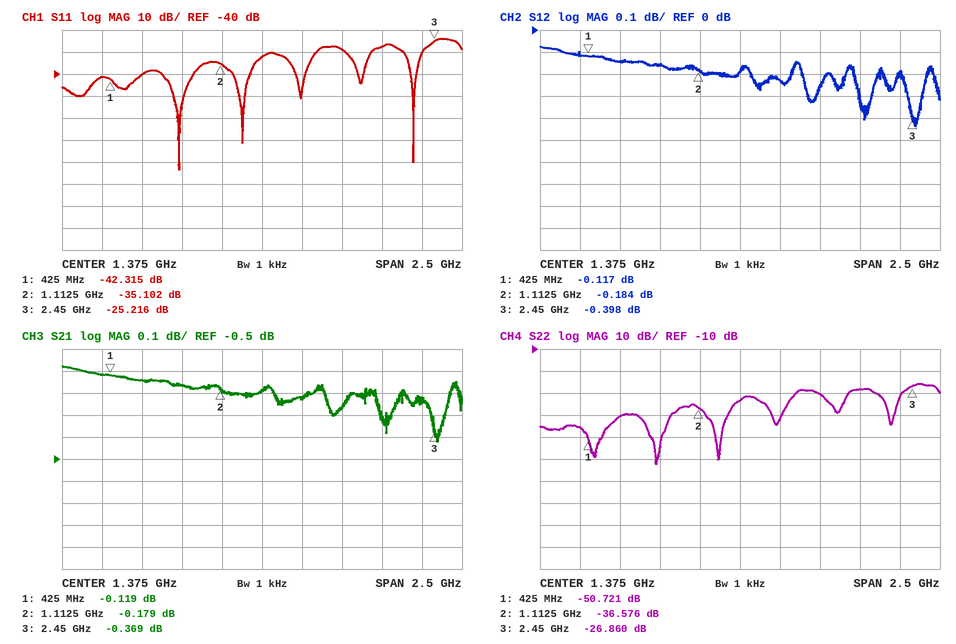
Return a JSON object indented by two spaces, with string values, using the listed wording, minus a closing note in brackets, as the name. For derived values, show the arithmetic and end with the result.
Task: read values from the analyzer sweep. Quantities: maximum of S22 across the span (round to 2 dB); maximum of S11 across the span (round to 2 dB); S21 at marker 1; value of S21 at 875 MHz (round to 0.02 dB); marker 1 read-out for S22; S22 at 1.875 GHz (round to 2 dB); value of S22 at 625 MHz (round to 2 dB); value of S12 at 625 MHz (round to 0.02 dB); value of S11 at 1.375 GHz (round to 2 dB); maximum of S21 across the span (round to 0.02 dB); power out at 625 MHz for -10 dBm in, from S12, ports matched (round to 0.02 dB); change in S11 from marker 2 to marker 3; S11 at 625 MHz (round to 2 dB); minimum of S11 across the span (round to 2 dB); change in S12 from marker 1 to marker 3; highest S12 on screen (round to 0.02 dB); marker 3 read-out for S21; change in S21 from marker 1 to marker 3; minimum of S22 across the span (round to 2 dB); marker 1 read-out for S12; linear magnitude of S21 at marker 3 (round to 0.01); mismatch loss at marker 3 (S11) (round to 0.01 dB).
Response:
{
  "maximum of S22 across the span": "-26 dB",
  "maximum of S11 across the span": "-24 dB",
  "S21 at marker 1": "-0.119 dB",
  "value of S21 at 875 MHz": "-0.16 dB",
  "marker 1 read-out for S22": "-50.721 dB",
  "S22 at 1.875 GHz": "-30 dB",
  "value of S22 at 625 MHz": "-40 dB",
  "value of S12 at 625 MHz": "-0.14 dB",
  "value of S11 at 1.375 GHz": "-32 dB",
  "maximum of S21 across the span": "-0.08 dB",
  "power out at 625 MHz for -10 dBm in, from S12, ports matched": "-10 dBm + (-0.14 dB) = -10.14 dBm",
  "change in S11 from marker 2 to marker 3": "-25.216 − (-35.102) = 9.886 dB",
  "S11 at 625 MHz": "-40 dB",
  "minimum of S11 across the span": "-84 dB",
  "change in S12 from marker 1 to marker 3": "-0.398 − (-0.117) = -0.281 dB",
  "highest S12 on screen": "-0.08 dB",
  "marker 3 read-out for S21": "-0.369 dB",
  "change in S21 from marker 1 to marker 3": "-0.369 − (-0.119) = -0.250 dB",
  "minimum of S22 across the span": "-62 dB",
  "marker 1 read-out for S12": "-0.117 dB",
  "linear magnitude of S21 at marker 3": "10^(-0.369/20) ≈ 0.96",
  "mismatch loss at marker 3 (S11)": "−10 log10(1 − 10^(-25.216/10)) ≈ 0.01 dB"
}
